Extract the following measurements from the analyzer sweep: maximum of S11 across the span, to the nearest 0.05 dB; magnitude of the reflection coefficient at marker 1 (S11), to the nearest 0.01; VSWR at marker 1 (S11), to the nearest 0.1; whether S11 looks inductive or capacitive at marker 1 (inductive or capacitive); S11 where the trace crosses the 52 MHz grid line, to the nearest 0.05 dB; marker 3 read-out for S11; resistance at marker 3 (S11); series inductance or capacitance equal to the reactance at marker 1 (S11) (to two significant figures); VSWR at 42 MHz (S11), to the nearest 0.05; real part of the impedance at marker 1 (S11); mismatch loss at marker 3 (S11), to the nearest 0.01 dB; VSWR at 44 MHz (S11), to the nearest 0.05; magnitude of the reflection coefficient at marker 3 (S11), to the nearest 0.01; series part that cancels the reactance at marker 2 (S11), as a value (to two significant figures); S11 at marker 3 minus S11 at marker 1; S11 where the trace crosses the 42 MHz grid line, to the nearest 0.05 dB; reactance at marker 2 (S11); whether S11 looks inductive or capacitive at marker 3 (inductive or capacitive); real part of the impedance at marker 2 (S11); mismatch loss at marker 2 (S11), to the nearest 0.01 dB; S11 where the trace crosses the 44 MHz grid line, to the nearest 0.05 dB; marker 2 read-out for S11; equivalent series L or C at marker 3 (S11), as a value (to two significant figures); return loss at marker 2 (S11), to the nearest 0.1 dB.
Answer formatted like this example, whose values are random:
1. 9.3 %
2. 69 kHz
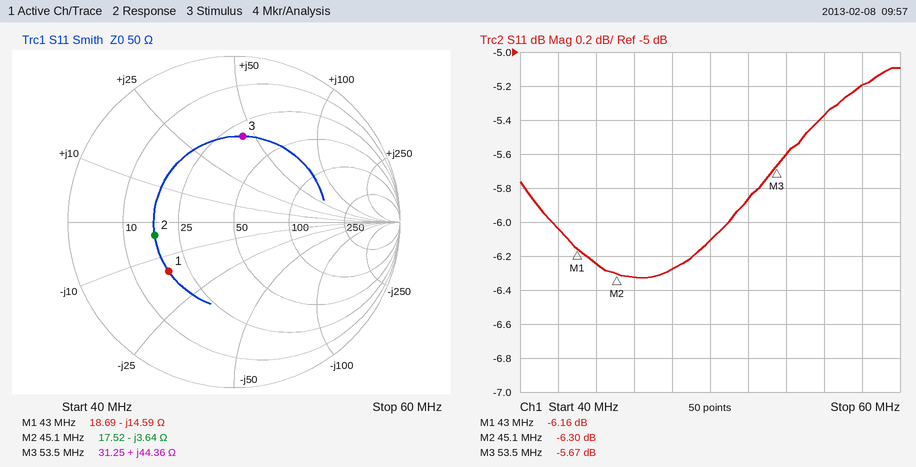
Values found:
1. -5.10 dB
2. 0.49
3. 2.9
4. capacitive
5. -5.85 dB
6. -5.67 dB
7. 31.25 Ω
8. 250 pF
9. 3.00
10. 18.69 Ω
11. 1.37 dB
12. 2.90
13. 0.52
14. 13 nH
15. 0.49 dB
16. -6.05 dB
17. -3.64 Ω
18. inductive
19. 17.52 Ω
20. 1.16 dB
21. -6.25 dB
22. -6.30 dB
23. 130 nH
24. 6.3 dB
